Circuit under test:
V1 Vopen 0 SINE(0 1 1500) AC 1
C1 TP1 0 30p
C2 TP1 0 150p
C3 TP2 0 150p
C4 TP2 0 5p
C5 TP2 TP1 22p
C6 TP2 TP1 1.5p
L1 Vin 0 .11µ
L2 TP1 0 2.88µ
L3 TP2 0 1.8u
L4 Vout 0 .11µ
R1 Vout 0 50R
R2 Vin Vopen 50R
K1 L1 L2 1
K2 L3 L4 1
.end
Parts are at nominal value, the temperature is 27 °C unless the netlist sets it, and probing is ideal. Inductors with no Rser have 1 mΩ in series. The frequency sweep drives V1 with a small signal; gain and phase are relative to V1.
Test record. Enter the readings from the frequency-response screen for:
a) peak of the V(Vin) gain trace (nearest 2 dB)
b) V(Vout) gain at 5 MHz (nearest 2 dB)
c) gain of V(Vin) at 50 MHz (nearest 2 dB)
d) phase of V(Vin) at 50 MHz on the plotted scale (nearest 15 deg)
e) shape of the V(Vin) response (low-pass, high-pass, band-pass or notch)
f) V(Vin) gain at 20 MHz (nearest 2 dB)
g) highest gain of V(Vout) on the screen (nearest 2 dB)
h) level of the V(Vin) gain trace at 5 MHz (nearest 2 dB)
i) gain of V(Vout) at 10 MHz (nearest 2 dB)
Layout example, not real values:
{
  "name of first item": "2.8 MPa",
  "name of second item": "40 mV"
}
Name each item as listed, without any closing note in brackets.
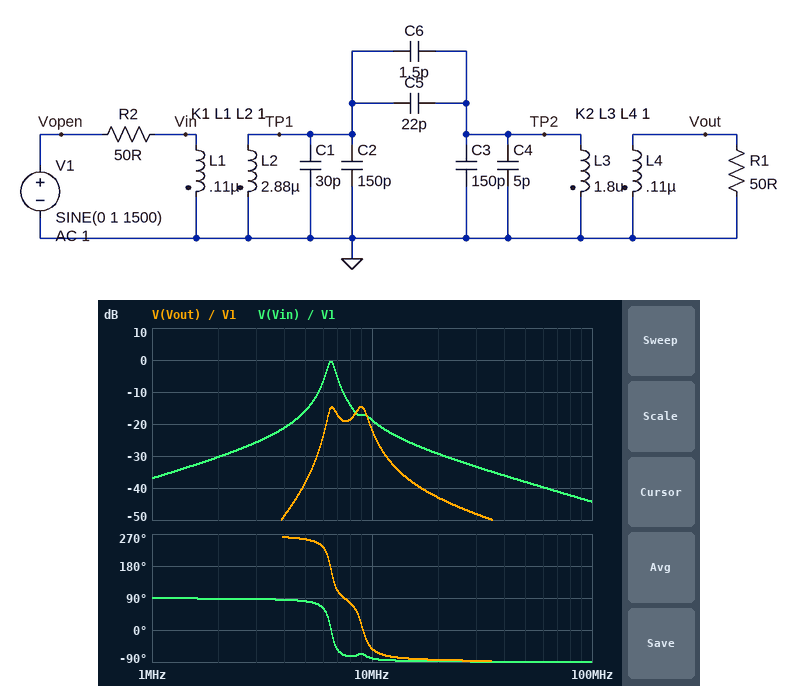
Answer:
{
  "peak of the V(Vin) gain trace": "0 dB",
  "V(Vout) gain at 5 MHz": "-38 dB",
  "gain of V(Vin) at 50 MHz": "-38 dB",
  "phase of V(Vin) at 50 MHz on the plotted scale": "-90 deg",
  "shape of the V(Vin) response": "band-pass",
  "V(Vin) gain at 20 MHz": "-30 dB",
  "highest gain of V(Vout) on the screen": "-14 dB",
  "level of the V(Vin) gain trace at 5 MHz": "-16 dB",
  "gain of V(Vout) at 10 MHz": "-22 dB"
}
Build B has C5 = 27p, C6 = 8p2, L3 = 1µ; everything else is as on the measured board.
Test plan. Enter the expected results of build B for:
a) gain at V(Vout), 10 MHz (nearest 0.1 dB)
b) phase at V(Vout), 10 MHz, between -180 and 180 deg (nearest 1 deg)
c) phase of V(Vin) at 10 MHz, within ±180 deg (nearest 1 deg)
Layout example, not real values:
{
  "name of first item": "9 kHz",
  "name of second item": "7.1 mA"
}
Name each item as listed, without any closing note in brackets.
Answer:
{
  "gain at V(Vout), 10 MHz": "-23.1 dB",
  "phase at V(Vout), 10 MHz, between -180 and 180 deg": "69 deg",
  "phase of V(Vin) at 10 MHz, within ±180 deg": "-82 deg"
}
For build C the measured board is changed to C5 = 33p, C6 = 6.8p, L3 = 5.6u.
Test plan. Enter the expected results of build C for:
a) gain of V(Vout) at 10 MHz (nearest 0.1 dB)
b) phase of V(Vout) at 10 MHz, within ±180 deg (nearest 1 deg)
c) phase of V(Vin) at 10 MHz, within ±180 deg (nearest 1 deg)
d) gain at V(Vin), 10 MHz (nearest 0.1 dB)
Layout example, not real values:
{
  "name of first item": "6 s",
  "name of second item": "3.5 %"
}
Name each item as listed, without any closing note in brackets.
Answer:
{
  "gain of V(Vout) at 10 MHz": "-34.4 dB",
  "phase of V(Vout) at 10 MHz, within ±180 deg": "-82 deg",
  "phase of V(Vin) at 10 MHz, within ±180 deg": "-84 deg",
  "gain at V(Vin), 10 MHz": "-20.0 dB"
}
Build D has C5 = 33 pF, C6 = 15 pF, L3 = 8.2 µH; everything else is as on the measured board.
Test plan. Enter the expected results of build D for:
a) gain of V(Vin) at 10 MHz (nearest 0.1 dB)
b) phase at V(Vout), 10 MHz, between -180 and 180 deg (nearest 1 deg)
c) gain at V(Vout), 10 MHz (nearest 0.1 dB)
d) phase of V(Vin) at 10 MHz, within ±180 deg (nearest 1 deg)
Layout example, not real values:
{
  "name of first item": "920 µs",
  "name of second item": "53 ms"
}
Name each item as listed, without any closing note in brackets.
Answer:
{
  "gain of V(Vin) at 10 MHz": "-20.4 dB",
  "phase at V(Vout), 10 MHz, between -180 and 180 deg": "-83 deg",
  "gain at V(Vout), 10 MHz": "-36.0 dB",
  "phase of V(Vin) at 10 MHz, within ±180 deg": "-84 deg"
}
